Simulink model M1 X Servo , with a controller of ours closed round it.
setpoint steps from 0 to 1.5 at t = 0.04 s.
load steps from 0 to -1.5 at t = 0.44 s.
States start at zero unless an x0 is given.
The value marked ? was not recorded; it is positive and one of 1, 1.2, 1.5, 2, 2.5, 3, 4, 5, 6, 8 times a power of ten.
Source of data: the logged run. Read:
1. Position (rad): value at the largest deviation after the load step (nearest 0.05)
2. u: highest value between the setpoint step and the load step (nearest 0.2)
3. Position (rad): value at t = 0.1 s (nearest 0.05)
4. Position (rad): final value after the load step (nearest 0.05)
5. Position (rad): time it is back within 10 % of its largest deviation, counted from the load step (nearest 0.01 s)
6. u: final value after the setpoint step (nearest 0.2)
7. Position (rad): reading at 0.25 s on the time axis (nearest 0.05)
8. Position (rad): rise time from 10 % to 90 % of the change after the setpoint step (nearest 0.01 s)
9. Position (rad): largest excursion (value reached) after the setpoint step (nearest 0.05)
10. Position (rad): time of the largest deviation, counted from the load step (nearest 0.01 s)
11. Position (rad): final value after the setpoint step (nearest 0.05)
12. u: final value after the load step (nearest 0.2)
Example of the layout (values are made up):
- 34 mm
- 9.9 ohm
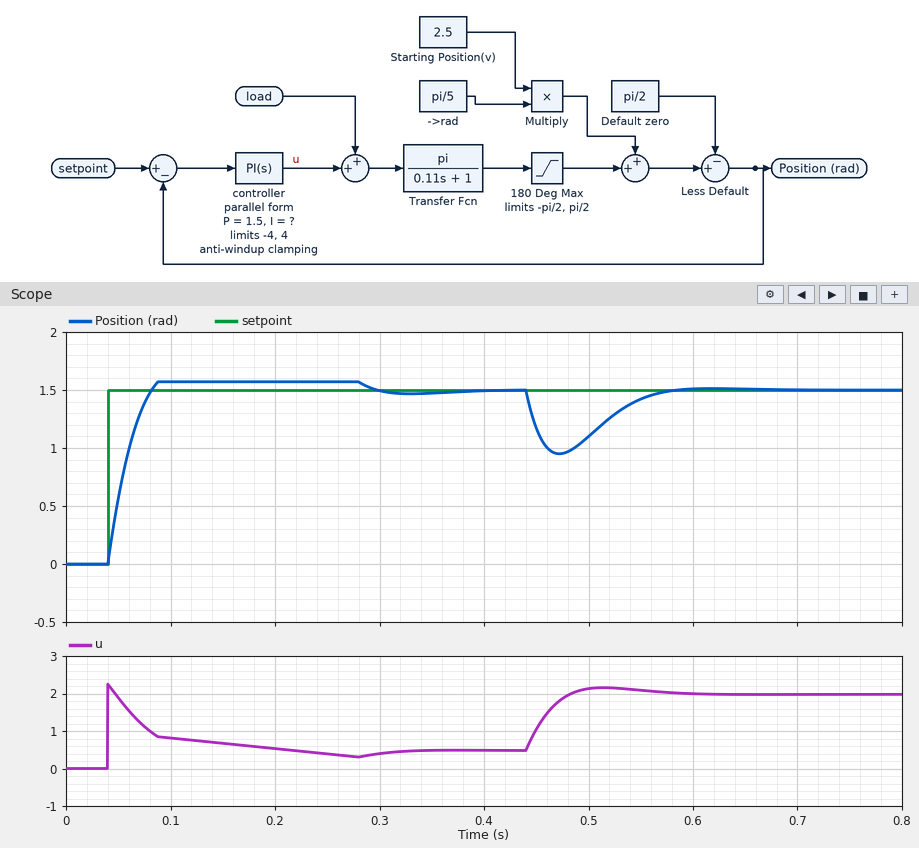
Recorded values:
- 0.95
- 2.2
- 1.55
- 1.50
- 0.12 s
- 0.4
- 1.55
- 0.03 s
- 1.55
- 0.03 s
- 1.50
- 2.0
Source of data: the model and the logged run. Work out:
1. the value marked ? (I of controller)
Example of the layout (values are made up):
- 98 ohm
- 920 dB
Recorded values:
- 40
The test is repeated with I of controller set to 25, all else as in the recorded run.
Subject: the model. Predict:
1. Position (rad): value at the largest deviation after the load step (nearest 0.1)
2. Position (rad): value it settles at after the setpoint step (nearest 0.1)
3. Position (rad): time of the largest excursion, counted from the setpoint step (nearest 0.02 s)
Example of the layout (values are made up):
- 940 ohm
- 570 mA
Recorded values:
- 0.9
- 1.5
- 0.08 s
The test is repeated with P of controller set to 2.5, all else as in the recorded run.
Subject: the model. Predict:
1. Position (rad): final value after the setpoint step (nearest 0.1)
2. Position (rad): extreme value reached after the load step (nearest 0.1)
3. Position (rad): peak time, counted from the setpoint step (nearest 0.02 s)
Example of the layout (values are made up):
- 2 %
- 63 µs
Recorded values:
- 1.5
- 1.1
- 0.06 s
